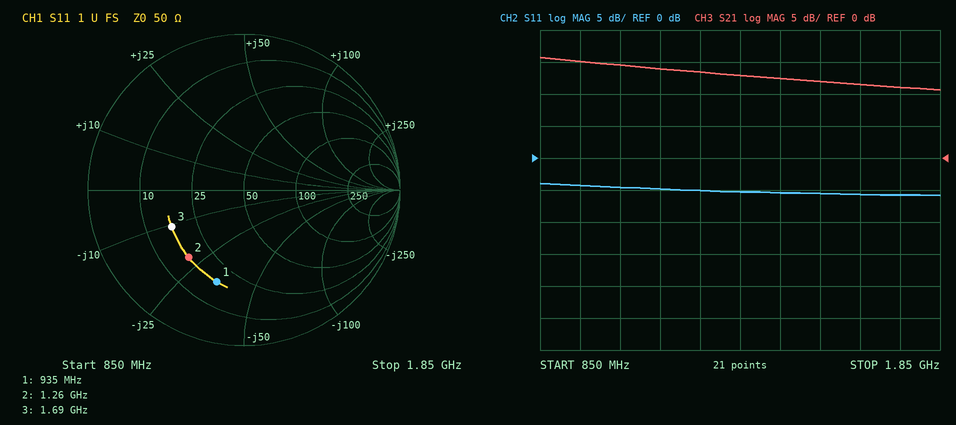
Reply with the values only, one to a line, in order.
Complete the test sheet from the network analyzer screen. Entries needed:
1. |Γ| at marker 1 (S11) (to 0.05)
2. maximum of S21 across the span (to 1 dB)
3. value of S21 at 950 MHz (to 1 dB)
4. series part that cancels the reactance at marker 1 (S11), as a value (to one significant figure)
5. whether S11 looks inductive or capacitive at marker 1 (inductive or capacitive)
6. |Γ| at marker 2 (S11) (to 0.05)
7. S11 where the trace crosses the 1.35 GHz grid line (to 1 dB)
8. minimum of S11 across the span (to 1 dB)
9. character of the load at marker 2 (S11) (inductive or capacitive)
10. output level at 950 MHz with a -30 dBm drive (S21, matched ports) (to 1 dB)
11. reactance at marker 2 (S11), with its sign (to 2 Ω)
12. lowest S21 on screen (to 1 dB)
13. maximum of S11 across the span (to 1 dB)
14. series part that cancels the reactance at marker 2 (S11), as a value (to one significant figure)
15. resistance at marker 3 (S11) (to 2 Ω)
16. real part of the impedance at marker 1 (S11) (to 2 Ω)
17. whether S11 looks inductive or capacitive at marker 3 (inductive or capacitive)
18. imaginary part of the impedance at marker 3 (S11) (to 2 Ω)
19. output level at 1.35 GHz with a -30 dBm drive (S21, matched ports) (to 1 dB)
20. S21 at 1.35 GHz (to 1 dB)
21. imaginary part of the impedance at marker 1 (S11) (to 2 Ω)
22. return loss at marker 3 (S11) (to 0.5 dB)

0.60
16 dB
15 dB
6 nH
capacitive
0.55
-5 dB
-6 dB
capacitive
-15 dBm
-22 Ω
11 dB
-4 dB
3 nH
16 Ω
18 Ω
capacitive
-10 Ω
-17 dBm
13 dB
-34 Ω
5.5 dB
